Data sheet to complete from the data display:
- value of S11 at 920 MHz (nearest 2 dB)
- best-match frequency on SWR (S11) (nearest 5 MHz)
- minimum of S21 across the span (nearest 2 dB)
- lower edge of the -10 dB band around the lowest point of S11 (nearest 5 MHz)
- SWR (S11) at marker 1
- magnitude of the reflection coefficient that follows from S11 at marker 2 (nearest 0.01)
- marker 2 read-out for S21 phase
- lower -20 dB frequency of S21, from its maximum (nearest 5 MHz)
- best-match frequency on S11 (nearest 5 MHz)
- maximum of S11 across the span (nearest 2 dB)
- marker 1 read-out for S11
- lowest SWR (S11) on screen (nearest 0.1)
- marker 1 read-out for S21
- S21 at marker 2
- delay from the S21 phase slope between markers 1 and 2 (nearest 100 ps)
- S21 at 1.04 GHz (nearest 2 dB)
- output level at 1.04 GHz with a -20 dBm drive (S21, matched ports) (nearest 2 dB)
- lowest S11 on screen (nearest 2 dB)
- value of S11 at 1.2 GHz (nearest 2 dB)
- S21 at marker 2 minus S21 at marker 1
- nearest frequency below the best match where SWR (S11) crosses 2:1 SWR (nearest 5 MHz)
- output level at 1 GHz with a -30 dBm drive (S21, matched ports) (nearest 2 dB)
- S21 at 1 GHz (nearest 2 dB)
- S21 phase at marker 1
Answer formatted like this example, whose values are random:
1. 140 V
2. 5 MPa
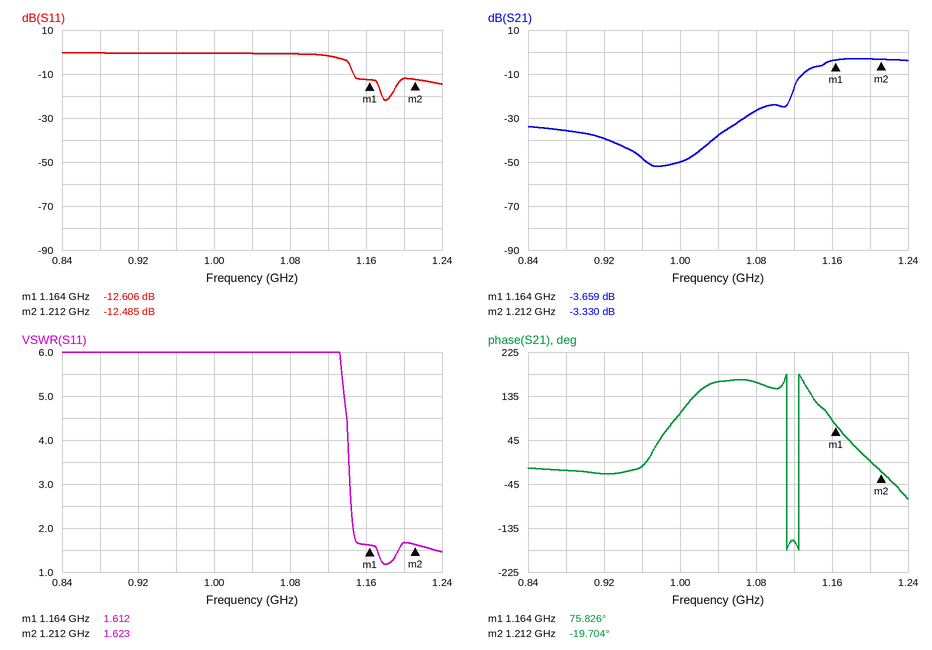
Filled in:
1. 0 dB
2. 1.180 GHz
3. -52 dB
4. 1.145 GHz
5. 1.612
6. 0.24
7. -19.704°
8. 1.115 GHz
9. 1.180 GHz
10. 0 dB
11. -12.606 dB
12. 1.2
13. -3.659 dB
14. -3.330 dB
15. 5.5 ns
16. -38 dB
17. -58 dBm
18. -22 dB
19. -12 dB
20. 0.329 dB
21. 1.145 GHz
22. -80 dBm
23. -50 dB
24. 75.826°
